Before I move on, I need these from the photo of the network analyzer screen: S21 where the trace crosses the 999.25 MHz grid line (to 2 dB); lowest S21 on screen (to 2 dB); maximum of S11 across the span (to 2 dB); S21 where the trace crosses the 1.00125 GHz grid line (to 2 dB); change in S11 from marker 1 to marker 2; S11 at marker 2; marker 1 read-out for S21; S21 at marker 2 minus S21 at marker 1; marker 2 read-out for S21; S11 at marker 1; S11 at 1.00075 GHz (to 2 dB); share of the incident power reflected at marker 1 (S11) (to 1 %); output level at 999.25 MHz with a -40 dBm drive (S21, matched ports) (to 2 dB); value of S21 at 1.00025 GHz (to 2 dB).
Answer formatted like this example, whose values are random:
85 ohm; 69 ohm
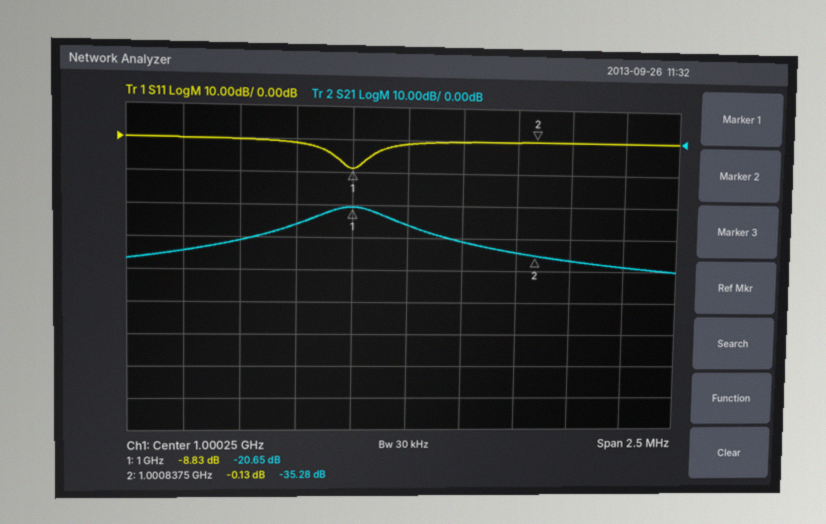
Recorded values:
-34 dB; -40 dB; 0 dB; -38 dB; 8.70 dB; -0.13 dB; -20.65 dB; -14.63 dB; -35.28 dB; -8.83 dB; 0 dB; 13 %; -74 dBm; -26 dB
